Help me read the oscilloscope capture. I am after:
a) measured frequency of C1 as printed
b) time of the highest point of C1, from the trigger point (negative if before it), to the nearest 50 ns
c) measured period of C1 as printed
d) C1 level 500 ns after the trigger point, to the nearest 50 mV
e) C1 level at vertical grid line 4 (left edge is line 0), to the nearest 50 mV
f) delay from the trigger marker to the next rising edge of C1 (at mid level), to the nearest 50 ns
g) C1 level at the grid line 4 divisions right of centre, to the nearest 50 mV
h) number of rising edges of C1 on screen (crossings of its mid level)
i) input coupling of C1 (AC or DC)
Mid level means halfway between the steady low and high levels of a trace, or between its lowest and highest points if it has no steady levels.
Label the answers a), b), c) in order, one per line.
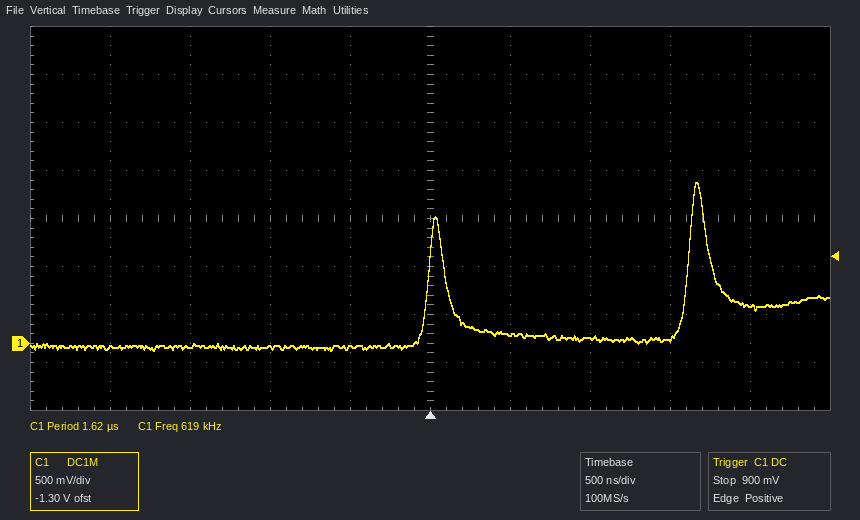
a) 619 kHz
b) +1.65 µs
c) 1.62 µs
d) 100 mV
e) -50 mV
f) 1.60 µs
g) 400 mV
h) 2
i) DC
